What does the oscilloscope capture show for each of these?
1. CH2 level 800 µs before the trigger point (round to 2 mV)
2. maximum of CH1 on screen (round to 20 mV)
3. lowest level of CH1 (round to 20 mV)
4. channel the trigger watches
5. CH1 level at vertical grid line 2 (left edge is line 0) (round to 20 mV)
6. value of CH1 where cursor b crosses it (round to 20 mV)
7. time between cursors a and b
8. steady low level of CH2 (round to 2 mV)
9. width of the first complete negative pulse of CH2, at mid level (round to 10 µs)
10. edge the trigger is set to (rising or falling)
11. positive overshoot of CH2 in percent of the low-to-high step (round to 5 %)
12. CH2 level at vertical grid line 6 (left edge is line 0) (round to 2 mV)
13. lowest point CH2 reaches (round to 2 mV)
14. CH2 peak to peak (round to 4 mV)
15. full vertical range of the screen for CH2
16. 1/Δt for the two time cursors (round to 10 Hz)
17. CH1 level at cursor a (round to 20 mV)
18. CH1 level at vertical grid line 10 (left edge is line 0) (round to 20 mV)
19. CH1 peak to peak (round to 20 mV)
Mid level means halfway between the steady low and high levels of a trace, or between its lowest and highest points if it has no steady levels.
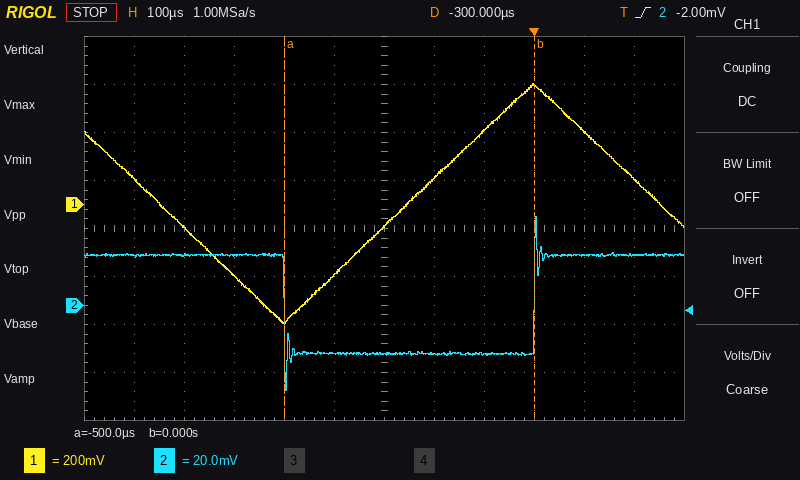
20 mV
500 mV
-500 mV
CH2
-100 mV
500 mV
500 µs
-20 mV
500 µs
rising
40 %
-20 mV
-36 mV
72 mV
160 mV
2.00 kHz
-480 mV
300 mV
1.00 V
